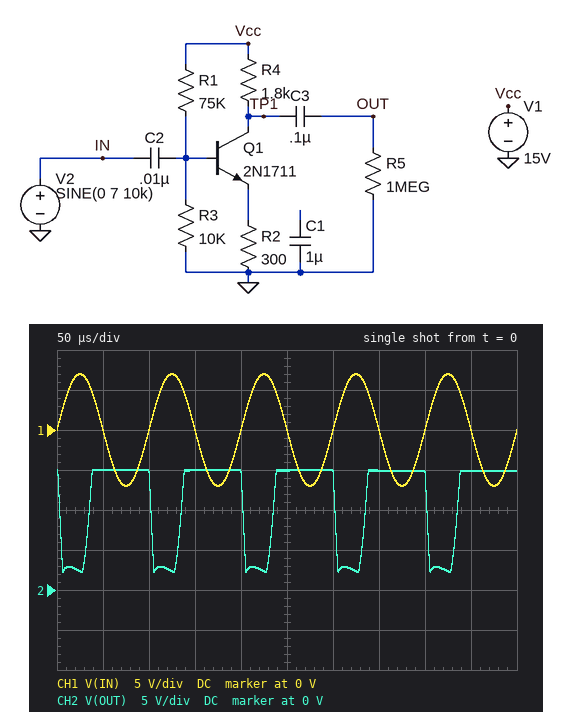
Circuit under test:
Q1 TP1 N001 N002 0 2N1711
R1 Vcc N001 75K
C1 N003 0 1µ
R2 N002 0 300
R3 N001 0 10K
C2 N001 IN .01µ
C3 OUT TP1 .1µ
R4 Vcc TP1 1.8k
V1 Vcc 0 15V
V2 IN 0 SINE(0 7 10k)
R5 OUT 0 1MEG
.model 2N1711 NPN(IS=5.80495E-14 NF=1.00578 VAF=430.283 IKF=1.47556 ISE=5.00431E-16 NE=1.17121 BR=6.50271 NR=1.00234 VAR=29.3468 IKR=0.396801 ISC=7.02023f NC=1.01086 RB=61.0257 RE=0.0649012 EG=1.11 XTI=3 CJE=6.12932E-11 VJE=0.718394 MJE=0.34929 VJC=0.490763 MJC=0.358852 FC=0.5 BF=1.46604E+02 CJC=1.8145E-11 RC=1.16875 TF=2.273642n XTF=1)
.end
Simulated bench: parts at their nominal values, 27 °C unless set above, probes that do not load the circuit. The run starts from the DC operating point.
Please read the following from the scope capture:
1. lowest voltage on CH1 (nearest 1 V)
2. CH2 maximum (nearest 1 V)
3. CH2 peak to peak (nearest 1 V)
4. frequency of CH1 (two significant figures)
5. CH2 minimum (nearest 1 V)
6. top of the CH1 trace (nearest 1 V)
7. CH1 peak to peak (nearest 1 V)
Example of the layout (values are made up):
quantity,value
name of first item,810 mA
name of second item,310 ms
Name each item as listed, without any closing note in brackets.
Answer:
quantity,value
lowest voltage on CH1,-7 V
CH2 maximum,15 V
CH2 peak to peak,13 V
frequency of CH1,10 kHz
CH2 minimum,2 V
top of the CH1 trace,7 V
CH1 peak to peak,14 V
